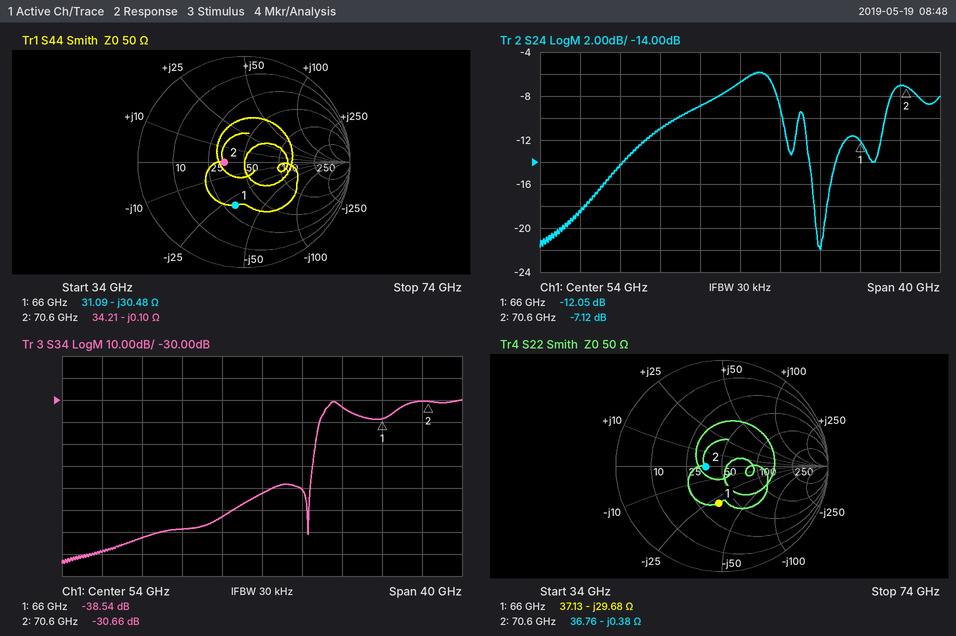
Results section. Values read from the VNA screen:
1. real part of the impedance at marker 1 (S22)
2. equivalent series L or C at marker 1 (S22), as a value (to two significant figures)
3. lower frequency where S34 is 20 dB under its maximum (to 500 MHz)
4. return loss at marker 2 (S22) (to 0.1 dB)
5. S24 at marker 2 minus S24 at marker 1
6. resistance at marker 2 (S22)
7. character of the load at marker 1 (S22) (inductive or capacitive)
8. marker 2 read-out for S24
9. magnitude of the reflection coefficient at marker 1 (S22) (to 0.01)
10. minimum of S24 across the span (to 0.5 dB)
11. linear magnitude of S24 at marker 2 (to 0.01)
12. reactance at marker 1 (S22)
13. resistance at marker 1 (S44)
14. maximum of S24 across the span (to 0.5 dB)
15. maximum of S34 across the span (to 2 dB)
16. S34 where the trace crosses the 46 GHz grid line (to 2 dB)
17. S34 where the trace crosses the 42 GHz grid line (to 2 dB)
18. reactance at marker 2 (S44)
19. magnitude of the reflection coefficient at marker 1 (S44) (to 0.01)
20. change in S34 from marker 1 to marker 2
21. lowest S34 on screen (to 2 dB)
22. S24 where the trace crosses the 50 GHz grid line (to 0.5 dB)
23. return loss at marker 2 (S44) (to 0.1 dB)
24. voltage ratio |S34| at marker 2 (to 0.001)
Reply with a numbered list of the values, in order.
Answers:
1. 37.13 Ω
2. 81 fF
3. 59.5 GHz
4. 16.3 dB
5. 4.93 dB
6. 36.76 Ω
7. capacitive
8. -7.12 dB
9. 0.35
10. -22.0 dB
11. 0.44
12. -29.68 Ω
13. 31.09 Ω
14. -6.0 dB
15. -30 dB
16. -88 dB
17. -92 dB
18. -0.10 Ω
19. 0.41
20. 7.88 dB
21. -104 dB
22. -9.0 dB
23. 14.5 dB
24. 0.029
